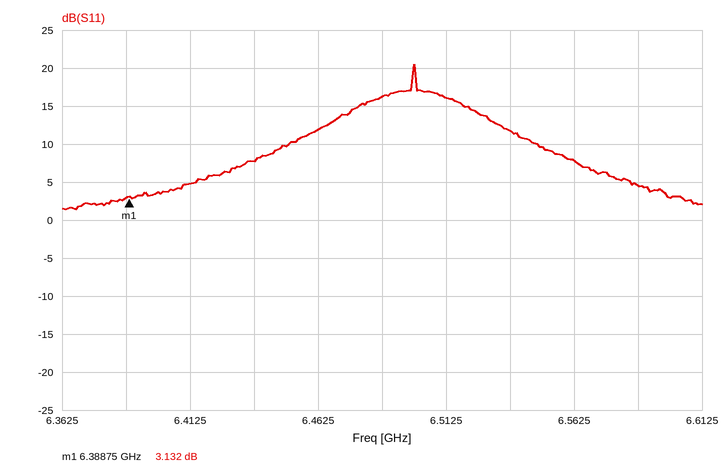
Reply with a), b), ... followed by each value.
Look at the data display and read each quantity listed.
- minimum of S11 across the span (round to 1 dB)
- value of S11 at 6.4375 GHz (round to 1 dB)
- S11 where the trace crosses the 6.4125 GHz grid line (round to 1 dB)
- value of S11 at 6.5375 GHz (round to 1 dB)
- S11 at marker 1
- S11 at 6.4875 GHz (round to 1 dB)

a) 1 dB
b) 8 dB
c) 5 dB
d) 12 dB
e) 3.132 dB
f) 16 dB
